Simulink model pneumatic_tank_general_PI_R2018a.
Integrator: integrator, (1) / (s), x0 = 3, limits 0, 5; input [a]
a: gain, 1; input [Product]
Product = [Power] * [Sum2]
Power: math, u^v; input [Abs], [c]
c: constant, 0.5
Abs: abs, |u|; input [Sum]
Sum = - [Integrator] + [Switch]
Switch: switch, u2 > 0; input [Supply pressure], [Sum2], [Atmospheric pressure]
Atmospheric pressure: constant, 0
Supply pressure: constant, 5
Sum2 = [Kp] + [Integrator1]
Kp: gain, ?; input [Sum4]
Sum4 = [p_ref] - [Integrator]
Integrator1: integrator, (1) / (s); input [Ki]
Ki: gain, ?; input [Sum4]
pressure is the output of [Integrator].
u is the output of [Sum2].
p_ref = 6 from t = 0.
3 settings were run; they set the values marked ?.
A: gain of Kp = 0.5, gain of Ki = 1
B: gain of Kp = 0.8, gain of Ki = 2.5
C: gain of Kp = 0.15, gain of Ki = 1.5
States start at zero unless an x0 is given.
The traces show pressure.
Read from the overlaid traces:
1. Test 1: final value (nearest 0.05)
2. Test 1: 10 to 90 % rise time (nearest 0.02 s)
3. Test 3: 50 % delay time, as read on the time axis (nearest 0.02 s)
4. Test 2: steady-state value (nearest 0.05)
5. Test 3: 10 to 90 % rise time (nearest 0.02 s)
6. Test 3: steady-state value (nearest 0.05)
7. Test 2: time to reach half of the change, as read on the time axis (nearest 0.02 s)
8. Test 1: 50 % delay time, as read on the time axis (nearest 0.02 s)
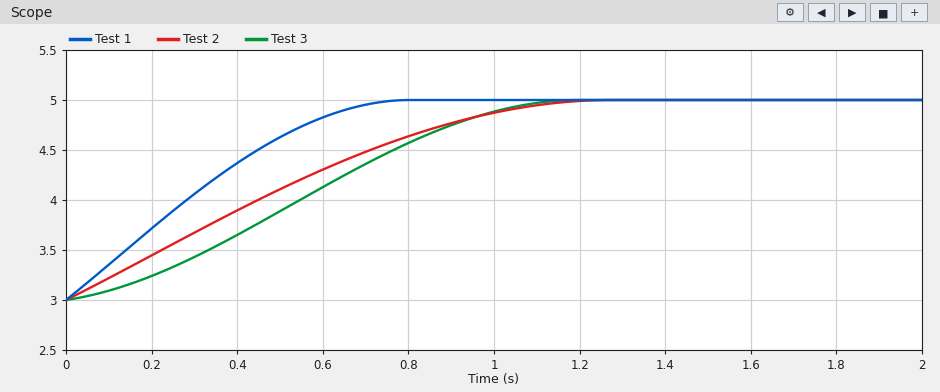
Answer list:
5.00
0.52 s
0.54 s
5.00
0.76 s
5.00
0.44 s
0.28 s
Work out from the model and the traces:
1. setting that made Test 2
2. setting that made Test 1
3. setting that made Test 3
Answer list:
A
B
C
